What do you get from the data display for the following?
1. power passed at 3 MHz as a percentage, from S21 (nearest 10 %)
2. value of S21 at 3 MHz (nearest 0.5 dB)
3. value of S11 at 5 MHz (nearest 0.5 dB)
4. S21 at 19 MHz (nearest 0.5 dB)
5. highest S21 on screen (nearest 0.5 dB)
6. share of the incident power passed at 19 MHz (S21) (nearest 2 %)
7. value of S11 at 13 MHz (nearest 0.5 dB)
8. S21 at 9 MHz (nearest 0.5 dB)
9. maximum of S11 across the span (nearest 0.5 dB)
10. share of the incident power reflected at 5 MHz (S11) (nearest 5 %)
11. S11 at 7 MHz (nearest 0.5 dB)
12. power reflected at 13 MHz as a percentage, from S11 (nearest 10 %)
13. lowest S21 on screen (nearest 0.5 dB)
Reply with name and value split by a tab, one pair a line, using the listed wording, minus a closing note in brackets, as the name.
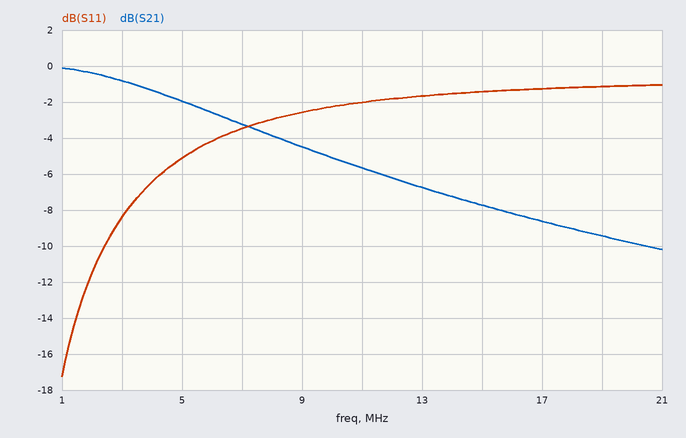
power passed at 3 MHz as a percentage, from S21	80 %
value of S21 at 3 MHz	-1.0 dB
value of S11 at 5 MHz	-5.0 dB
S21 at 19 MHz	-9.5 dB
highest S21 on screen	0.0 dB
share of the incident power passed at 19 MHz (S21)	12 %
value of S11 at 13 MHz	-1.5 dB
S21 at 9 MHz	-4.5 dB
maximum of S11 across the span	-1.0 dB
share of the incident power reflected at 5 MHz (S11)	30 %
S11 at 7 MHz	-3.5 dB
power reflected at 13 MHz as a percentage, from S11	70 %
lowest S21 on screen	-10.0 dB
